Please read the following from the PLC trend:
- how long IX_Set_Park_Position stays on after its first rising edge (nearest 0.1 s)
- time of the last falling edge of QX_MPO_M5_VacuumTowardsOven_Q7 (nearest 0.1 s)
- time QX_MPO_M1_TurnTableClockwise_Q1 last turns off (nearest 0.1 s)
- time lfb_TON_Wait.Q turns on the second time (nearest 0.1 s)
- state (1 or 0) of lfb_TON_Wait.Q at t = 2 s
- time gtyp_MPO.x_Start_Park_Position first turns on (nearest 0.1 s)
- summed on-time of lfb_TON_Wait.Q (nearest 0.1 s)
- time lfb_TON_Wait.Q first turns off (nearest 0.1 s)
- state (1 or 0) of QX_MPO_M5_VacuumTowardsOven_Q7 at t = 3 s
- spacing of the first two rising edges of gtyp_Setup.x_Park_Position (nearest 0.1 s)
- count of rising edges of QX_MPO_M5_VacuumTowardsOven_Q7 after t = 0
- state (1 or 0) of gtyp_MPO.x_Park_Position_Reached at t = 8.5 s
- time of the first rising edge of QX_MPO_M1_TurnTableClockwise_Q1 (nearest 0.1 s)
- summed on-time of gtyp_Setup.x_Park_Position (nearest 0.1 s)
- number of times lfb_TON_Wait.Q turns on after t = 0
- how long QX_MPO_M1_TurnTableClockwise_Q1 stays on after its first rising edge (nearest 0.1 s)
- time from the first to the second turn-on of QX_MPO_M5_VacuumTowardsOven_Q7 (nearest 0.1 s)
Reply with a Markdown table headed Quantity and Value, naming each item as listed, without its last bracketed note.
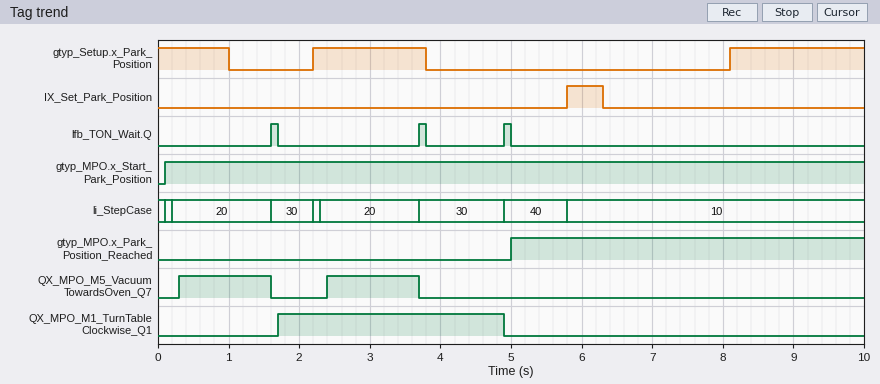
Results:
| Quantity | Value |
|---|---|
| how long IX_Set_Park_Position stays on after its first rising edge | 0.5 s |
| time of the last falling edge of QX_MPO_M5_VacuumTowardsOven_Q7 | 3.7 s |
| time QX_MPO_M1_TurnTableClockwise_Q1 last turns off | 4.9 s |
| time lfb_TON_Wait.Q turns on the second time | 3.7 s |
| state (1 or 0) of lfb_TON_Wait.Q at t = 2 s | 0 |
| time gtyp_MPO.x_Start_Park_Position first turns on | 0.1 s |
| summed on-time of lfb_TON_Wait.Q | 0.3 s |
| time lfb_TON_Wait.Q first turns off | 1.7 s |
| state (1 or 0) of QX_MPO_M5_VacuumTowardsOven_Q7 at t = 3 s | 1 |
| spacing of the first two rising edges of gtyp_Setup.x_Park_Position | 5.9 s |
| count of rising edges of QX_MPO_M5_VacuumTowardsOven_Q7 after t = 0 | 2 |
| state (1 or 0) of gtyp_MPO.x_Park_Position_Reached at t = 8.5 s | 1 |
| time of the first rising edge of QX_MPO_M1_TurnTableClockwise_Q1 | 1.7 s |
| summed on-time of gtyp_Setup.x_Park_Position | 4.5 s |
| number of times lfb_TON_Wait.Q turns on after t = 0 | 3 |
| how long QX_MPO_M1_TurnTableClockwise_Q1 stays on after its first rising edge | 3.2 s |
| time from the first to the second turn-on of QX_MPO_M5_VacuumTowardsOven_Q7 | 2.1 s |
